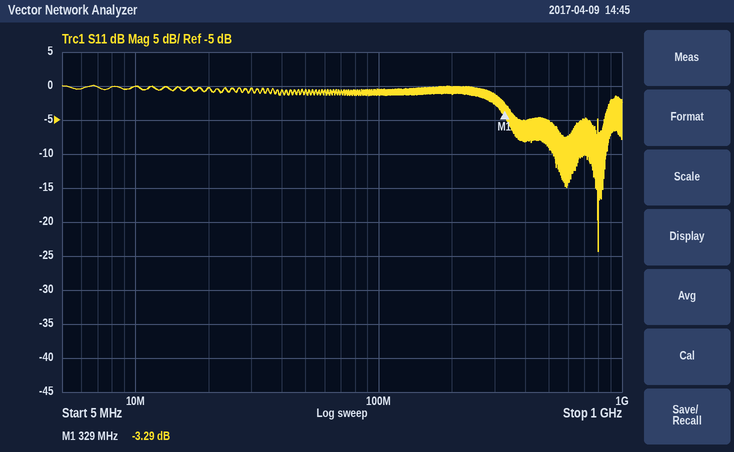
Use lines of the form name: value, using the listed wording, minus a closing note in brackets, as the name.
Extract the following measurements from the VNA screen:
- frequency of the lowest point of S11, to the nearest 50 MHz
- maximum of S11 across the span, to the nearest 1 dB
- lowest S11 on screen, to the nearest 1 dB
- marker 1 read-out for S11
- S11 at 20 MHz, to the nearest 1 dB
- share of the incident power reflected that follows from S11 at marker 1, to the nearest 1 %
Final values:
frequency of the lowest point of S11, to the nearest 50 MHz: 800 MHz
maximum of S11 across the span, to the nearest 1 dB: 0 dB
lowest S11 on screen, to the nearest 1 dB: -24 dB
marker 1 read-out for S11: -3.29 dB
S11 at 20 MHz, to the nearest 1 dB: 0 dB
share of the incident power reflected that follows from S11 at marker 1, to the nearest 1 %: 47 %
